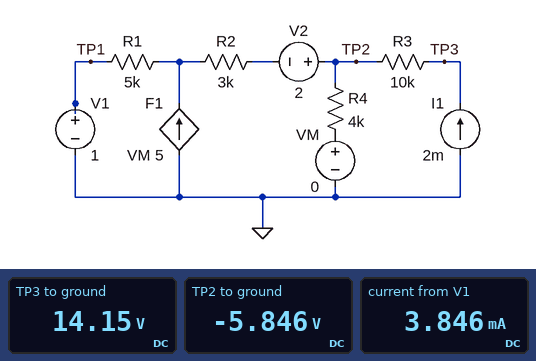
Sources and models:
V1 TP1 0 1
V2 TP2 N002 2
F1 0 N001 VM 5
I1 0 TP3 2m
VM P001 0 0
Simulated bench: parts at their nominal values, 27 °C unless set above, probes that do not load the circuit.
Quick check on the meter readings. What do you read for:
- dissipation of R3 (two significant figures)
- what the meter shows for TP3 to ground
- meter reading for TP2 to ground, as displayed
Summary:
40 mW
14.15 V
-5.846 V
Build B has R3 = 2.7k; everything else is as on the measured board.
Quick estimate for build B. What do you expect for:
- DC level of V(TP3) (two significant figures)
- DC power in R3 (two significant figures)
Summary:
-450 mV
11 mW
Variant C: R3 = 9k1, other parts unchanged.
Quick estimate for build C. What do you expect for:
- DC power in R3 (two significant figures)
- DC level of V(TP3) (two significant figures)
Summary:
36 mW
12 V
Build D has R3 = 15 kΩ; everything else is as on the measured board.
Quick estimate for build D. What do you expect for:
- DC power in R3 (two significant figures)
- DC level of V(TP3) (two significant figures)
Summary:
60 mW
24 V
